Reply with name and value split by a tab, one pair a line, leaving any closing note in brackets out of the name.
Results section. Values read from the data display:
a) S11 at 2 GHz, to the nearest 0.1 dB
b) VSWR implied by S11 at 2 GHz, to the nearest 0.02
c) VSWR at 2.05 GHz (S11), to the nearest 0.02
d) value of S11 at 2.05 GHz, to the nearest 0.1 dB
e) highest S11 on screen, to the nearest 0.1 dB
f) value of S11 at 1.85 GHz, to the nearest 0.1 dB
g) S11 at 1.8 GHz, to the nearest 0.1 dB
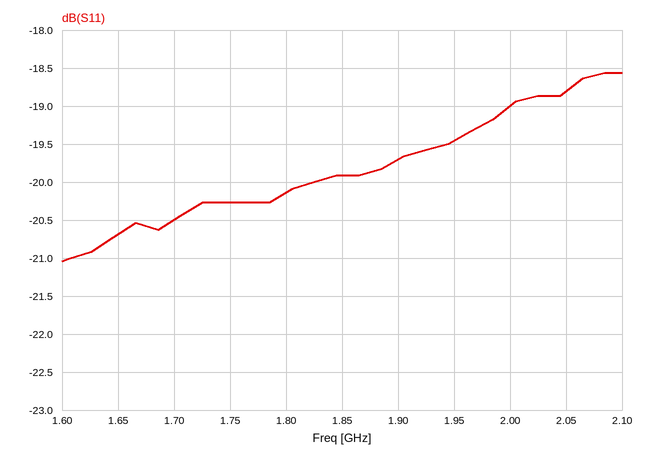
S11 at 2 GHz, to the nearest 0.1 dB	-19.0 dB
VSWR implied by S11 at 2 GHz, to the nearest 0.02	1.26
VSWR at 2.05 GHz (S11), to the nearest 0.02	1.26
value of S11 at 2.05 GHz, to the nearest 0.1 dB	-18.8 dB
highest S11 on screen, to the nearest 0.1 dB	-18.6 dB
value of S11 at 1.85 GHz, to the nearest 0.1 dB	-19.9 dB
S11 at 1.8 GHz, to the nearest 0.1 dB	-20.1 dB
